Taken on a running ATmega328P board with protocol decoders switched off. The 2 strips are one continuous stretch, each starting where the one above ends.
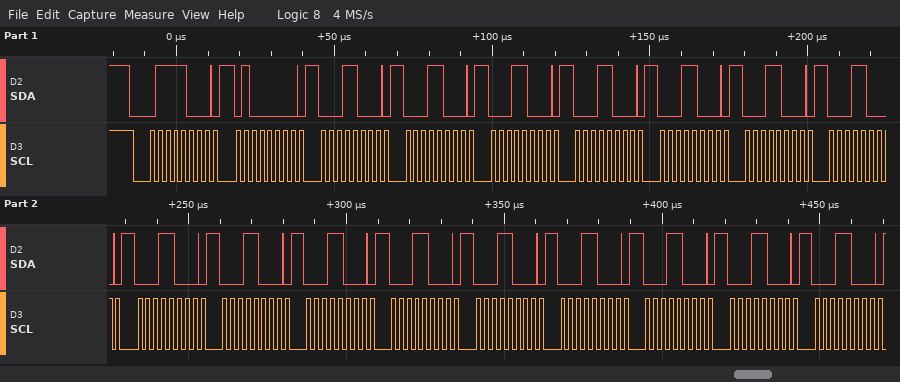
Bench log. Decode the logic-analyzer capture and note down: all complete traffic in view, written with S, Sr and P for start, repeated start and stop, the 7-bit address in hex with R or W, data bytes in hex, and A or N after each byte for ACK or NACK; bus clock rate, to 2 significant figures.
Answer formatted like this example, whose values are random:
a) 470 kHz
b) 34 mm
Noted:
a) S 3CW A 40 A 18 A 18 A 18 A 18 A 18 A 18 A 18 A 18 A 18 A 18 A 18 A 18 A 18 A 18 A 18 A 18 A
b) 400 kHz
